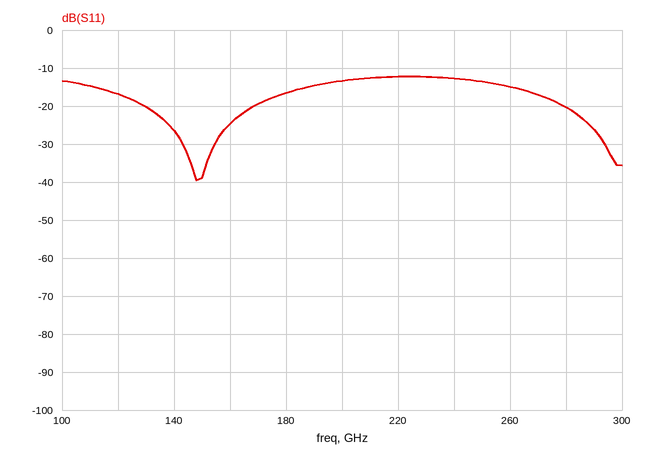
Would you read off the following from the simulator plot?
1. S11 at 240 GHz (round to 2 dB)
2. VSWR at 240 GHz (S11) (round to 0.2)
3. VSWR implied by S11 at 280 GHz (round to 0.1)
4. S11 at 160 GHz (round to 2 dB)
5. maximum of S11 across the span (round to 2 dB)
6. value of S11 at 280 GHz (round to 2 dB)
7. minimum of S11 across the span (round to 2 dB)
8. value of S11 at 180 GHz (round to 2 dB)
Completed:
-12 dB
1.6
1.2
-24 dB
-12 dB
-20 dB
-40 dB
-16 dB
